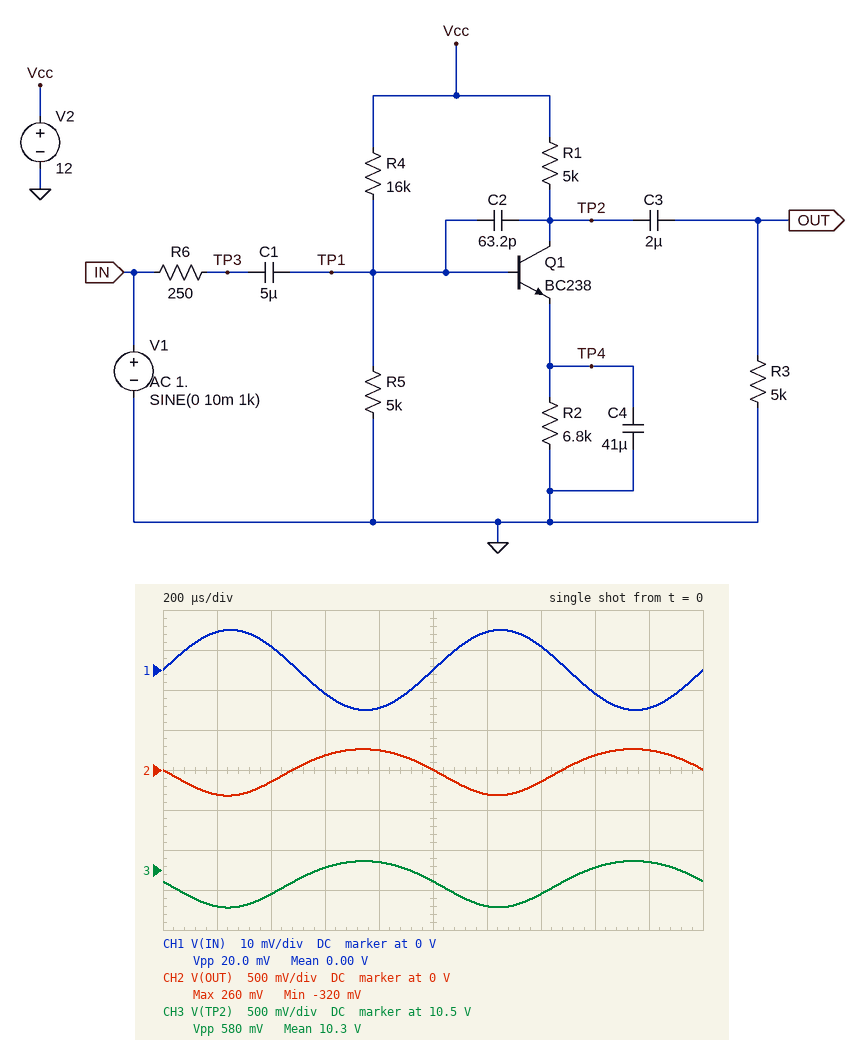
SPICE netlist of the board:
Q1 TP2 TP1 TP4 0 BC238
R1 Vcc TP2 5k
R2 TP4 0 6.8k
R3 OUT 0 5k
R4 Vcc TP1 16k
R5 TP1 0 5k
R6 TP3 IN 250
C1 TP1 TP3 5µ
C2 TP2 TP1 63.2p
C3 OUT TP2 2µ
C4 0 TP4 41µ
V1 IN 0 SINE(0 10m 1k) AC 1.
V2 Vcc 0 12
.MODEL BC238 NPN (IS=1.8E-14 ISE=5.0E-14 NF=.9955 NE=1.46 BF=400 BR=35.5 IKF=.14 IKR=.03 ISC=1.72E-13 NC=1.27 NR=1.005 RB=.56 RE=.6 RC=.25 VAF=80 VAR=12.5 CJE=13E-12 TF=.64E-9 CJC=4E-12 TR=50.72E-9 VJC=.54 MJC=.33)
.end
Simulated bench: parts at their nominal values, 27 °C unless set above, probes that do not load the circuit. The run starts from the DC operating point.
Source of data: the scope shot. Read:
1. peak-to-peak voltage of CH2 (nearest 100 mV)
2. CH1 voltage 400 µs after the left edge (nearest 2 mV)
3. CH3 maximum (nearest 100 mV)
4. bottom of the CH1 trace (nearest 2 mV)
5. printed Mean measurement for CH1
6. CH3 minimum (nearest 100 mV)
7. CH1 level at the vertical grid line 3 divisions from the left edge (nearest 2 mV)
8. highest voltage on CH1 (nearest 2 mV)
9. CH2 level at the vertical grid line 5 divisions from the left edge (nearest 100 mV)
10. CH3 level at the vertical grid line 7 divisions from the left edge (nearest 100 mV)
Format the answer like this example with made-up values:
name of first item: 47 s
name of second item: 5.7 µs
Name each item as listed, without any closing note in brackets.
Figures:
peak-to-peak voltage of CH2: 600 mV
CH1 voltage 400 µs after the left edge: 6 mV
CH3 maximum: 10.6 V
bottom of the CH1 trace: -10 mV
printed Mean measurement for CH1: 0.00 V
CH3 minimum: 10.0 V
CH1 level at the vertical grid line 3 divisions from the left edge: -6 mV
highest voltage on CH1: 10 mV
CH2 level at the vertical grid line 5 divisions from the left edge: 0 V
CH3 level at the vertical grid line 7 divisions from the left edge: 10.2 V
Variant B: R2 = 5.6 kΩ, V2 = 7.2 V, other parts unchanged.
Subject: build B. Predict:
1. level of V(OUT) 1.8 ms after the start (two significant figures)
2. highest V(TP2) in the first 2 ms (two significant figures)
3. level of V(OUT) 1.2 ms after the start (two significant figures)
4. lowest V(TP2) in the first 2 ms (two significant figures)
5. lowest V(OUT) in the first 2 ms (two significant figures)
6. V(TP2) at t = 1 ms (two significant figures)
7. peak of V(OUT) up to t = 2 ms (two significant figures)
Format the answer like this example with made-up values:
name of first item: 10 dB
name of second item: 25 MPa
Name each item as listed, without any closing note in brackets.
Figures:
level of V(OUT) 1.8 ms after the start: 150 mV
highest V(TP2) in the first 2 ms: 6.4 V
level of V(OUT) 1.2 ms after the start: -190 mV
lowest V(TP2) in the first 2 ms: 6.0 V
lowest V(OUT) in the first 2 ms: -200 mV
V(TP2) at t = 1 ms: 6.2 V
peak of V(OUT) up to t = 2 ms: 160 mV
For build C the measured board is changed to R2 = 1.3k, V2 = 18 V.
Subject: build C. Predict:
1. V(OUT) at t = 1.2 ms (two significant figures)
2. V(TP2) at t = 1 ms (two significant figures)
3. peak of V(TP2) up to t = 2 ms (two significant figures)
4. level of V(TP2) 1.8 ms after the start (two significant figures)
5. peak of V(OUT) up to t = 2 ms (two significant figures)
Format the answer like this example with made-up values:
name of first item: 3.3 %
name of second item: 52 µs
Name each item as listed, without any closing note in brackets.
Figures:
V(OUT) at t = 1.2 ms: -640 mV
V(TP2) at t = 1 ms: 3.8 V
peak of V(TP2) up to t = 2 ms: 6.0 V
level of V(TP2) 1.8 ms after the start: 5.6 V
peak of V(OUT) up to t = 2 ms: 1.7 V
